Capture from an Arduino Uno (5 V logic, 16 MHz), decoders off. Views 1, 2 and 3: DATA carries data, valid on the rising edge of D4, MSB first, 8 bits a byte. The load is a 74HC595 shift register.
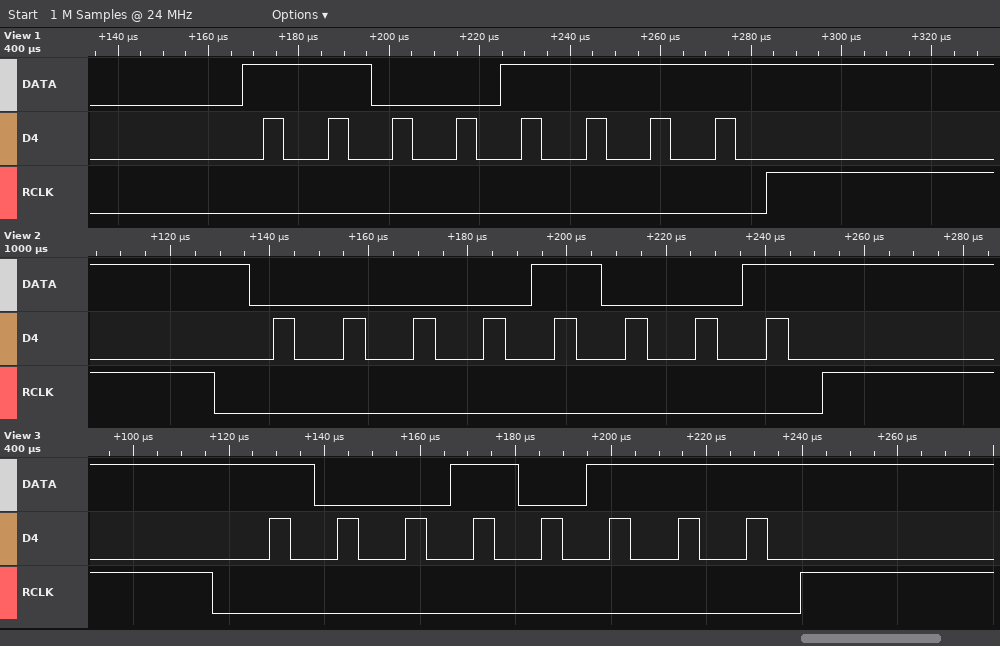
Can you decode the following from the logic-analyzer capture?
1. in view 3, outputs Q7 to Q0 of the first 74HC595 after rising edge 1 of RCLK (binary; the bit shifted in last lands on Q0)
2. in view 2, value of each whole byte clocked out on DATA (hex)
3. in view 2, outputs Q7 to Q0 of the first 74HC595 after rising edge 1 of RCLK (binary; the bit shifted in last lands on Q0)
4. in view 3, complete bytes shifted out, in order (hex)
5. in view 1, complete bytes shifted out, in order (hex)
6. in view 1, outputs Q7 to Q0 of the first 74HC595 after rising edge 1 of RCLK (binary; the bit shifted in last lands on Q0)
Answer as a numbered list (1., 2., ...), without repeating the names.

1. 10010111
2. 09
3. 00001001
4. 97
5. CF
6. 11001111
